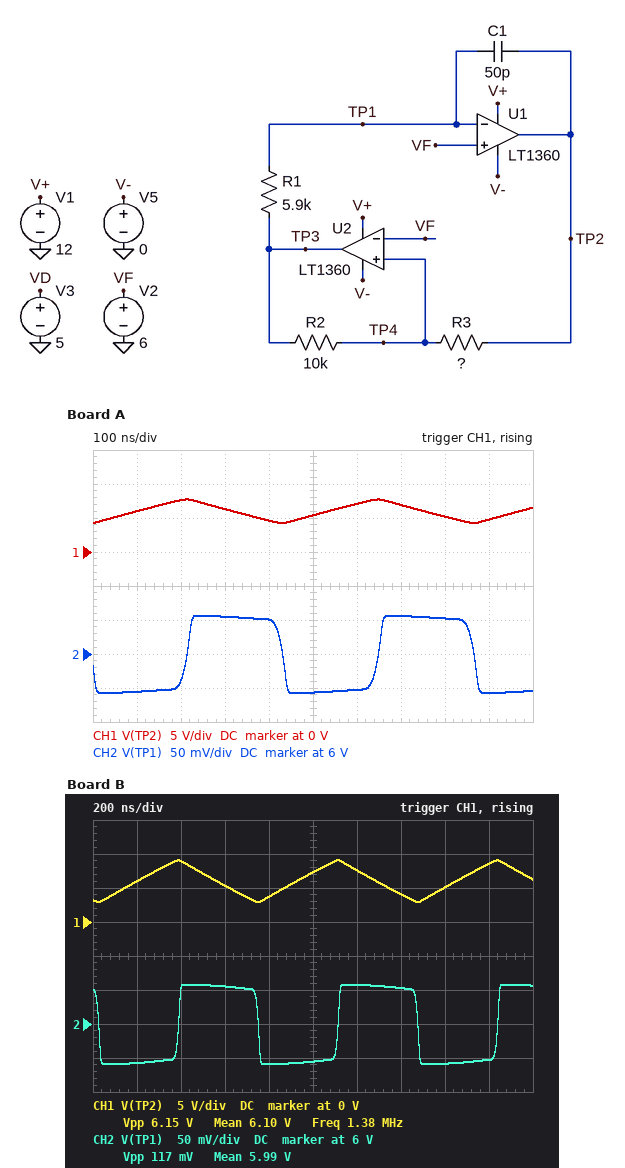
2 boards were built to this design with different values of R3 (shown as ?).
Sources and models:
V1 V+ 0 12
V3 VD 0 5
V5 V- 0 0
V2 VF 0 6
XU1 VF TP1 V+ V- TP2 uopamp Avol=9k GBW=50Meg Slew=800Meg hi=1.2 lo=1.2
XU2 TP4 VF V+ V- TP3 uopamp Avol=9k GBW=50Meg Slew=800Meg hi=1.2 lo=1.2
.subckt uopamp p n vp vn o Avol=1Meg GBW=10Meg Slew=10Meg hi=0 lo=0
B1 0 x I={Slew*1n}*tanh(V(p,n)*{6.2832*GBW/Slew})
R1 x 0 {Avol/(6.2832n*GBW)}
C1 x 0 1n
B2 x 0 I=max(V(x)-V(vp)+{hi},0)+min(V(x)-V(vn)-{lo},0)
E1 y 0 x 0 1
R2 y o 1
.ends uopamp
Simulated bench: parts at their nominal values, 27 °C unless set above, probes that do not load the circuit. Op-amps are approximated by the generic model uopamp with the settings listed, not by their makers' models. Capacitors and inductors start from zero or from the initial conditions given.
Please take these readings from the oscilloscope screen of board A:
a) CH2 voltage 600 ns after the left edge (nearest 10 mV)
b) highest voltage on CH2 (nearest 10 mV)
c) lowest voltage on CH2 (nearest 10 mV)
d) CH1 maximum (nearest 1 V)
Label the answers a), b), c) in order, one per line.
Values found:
a) 5.95 V
b) 6.06 V
c) 5.94 V
d) 8 V
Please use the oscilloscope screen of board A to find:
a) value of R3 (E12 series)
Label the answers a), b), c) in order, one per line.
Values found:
a) 2.7 kΩ
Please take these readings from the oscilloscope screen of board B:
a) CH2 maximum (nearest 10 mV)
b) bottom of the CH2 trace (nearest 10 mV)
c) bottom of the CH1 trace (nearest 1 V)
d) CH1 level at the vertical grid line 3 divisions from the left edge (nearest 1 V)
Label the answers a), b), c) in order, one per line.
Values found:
a) 6.06 V
b) 5.94 V
c) 3 V
d) 5 V
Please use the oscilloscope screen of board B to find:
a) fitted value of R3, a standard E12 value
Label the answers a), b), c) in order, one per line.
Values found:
a) 5.6 kΩ
